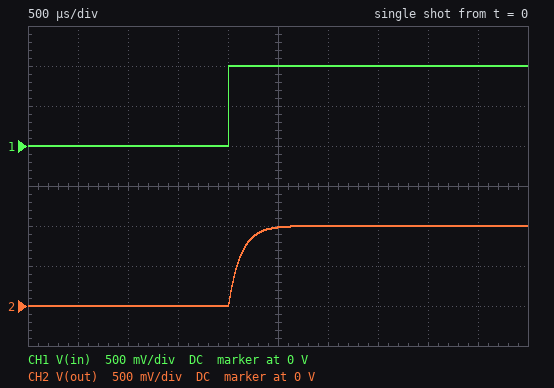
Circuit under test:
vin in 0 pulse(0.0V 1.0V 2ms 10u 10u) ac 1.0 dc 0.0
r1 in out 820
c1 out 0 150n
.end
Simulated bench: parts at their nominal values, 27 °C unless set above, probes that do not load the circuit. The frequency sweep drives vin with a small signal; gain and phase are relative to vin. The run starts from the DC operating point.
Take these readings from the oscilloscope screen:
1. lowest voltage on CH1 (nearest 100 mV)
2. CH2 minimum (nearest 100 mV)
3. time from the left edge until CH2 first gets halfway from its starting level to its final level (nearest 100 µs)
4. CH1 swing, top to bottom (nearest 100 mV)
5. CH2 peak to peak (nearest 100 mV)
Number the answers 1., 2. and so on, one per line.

1. 0 V
2. 0 V
3. 2.1 ms
4. 1.0 V
5. 1.0 V
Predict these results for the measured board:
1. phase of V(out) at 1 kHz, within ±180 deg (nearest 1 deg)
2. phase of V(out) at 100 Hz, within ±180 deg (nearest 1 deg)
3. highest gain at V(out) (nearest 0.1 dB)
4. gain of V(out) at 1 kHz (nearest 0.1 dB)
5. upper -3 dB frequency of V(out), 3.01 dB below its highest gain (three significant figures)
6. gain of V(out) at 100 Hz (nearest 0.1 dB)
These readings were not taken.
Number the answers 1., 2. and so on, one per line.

1. -38 deg
2. -4 deg
3. 0 dB
4. -2.0 dB
5. 1.29 kHz
6. 0 dB
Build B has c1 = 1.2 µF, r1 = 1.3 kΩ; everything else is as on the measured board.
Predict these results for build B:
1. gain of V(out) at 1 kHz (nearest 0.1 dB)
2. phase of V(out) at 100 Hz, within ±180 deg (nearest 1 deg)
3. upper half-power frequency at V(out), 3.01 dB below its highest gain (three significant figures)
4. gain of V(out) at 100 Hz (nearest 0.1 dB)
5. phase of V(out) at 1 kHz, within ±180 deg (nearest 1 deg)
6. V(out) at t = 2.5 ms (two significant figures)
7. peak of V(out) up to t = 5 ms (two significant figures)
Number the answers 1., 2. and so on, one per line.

1. -19.9 dB
2. -44 deg
3. 102 Hz
4. -2.9 dB
5. -84 deg
6. 270 mV
7. 850 mV
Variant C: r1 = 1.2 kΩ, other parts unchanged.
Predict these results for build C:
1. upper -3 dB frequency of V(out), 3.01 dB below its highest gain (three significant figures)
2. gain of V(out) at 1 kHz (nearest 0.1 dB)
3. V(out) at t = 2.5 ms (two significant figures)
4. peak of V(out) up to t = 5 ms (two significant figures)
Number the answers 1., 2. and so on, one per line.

1. 884 Hz
2. -3.6 dB
3. 940 mV
4. 1.0 V
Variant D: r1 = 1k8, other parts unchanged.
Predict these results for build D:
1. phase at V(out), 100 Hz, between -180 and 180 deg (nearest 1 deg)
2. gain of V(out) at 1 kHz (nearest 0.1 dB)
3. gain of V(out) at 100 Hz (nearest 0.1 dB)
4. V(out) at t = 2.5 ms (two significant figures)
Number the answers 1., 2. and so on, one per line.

1. -10 deg
2. -5.9 dB
3. -0.1 dB
4. 840 mV
